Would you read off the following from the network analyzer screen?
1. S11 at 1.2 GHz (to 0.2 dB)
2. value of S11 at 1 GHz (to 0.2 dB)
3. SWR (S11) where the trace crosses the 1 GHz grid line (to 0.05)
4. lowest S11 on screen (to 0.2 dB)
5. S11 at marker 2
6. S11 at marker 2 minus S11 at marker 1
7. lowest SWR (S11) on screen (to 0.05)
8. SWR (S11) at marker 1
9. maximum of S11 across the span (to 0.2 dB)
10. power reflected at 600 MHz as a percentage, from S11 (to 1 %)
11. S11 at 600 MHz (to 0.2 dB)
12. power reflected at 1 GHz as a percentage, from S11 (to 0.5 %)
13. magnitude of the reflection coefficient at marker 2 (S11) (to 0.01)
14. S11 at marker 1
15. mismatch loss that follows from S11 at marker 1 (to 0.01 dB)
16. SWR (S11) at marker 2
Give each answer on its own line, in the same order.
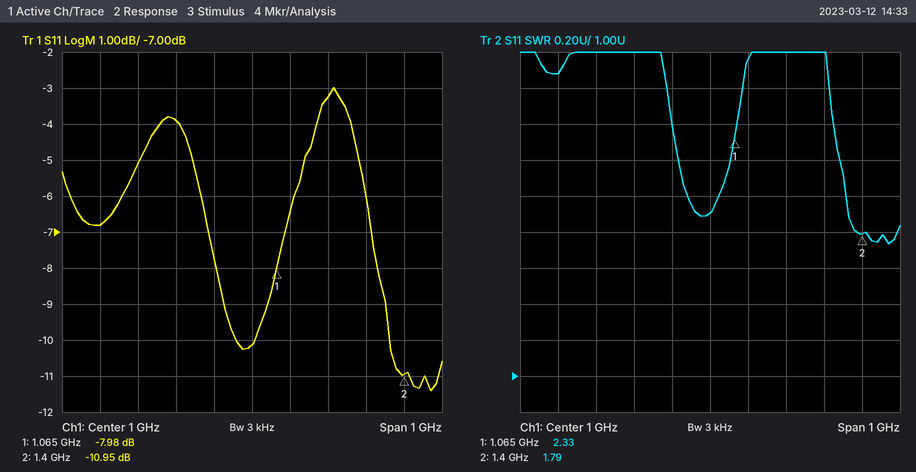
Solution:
-3.2 dB
-10.2 dB
1.90
-11.4 dB
-10.95 dB
-2.97 dB
1.75
2.33
-3.0 dB
21 %
-6.8 dB
9.5 %
0.28
-7.98 dB
0.75 dB
1.79
